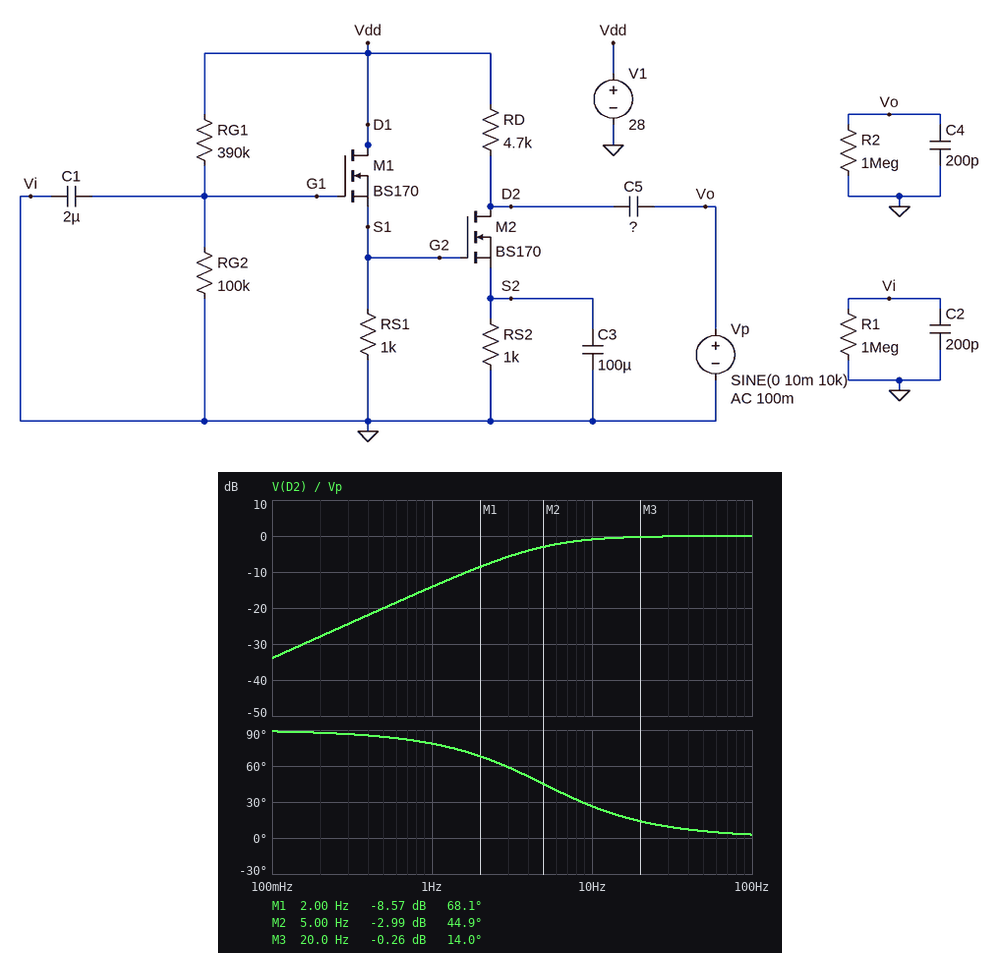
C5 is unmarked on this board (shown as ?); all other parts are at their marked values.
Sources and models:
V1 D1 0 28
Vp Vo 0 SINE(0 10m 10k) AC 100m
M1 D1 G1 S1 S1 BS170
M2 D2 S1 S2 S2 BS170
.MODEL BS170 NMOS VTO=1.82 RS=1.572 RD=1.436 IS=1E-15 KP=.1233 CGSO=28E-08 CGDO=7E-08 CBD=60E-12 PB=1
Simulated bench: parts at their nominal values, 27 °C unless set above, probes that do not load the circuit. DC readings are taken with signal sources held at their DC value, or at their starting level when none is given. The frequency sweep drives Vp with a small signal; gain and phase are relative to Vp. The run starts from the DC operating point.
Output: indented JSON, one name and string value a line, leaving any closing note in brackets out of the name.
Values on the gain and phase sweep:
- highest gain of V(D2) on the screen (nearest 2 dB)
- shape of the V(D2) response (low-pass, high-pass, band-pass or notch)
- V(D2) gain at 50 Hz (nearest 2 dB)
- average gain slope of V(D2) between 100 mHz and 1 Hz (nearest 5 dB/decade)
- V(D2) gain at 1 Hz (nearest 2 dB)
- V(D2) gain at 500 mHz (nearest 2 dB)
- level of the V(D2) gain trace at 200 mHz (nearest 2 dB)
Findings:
{
  "highest gain of V(D2) on the screen": "0 dB",
  "shape of the V(D2) response": "high-pass",
  "V(D2) gain at 50 Hz": "0 dB",
  "average gain slope of V(D2) between 100 mHz and 1 Hz": "20 dB/decade",
  "V(D2) gain at 1 Hz": "-14 dB",
  "V(D2) gain at 500 mHz": "-20 dB",
  "level of the V(D2) gain trace at 200 mHz": "-28 dB"
}
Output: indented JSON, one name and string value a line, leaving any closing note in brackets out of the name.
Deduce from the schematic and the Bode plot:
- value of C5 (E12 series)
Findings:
{
  "value of C5": "6.8 µF"
}
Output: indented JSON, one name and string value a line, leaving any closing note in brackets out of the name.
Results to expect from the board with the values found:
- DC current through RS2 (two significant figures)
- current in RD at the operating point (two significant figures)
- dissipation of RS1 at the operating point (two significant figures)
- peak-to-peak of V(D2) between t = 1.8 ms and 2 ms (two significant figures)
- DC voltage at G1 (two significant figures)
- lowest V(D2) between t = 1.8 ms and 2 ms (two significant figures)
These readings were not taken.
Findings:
{
  "DC current through RS2": "1.7 mA",
  "current in RD at the operating point": "1.7 mA",
  "dissipation of RS1 at the operating point": "13 mW",
  "peak-to-peak of V(D2) between t = 1.8 ms and 2 ms": "20 mV",
  "DC voltage at G1": "5.7 V",
  "lowest V(D2) between t = 1.8 ms and 2 ms": "20 V"
}
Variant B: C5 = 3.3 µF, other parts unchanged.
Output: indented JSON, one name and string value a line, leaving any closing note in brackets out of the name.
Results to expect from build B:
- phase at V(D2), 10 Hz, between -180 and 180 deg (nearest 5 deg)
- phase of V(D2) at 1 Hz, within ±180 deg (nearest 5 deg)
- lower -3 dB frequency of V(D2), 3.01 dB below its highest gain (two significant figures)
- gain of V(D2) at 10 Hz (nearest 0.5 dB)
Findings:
{
  "phase at V(D2), 10 Hz, between -180 and 180 deg": "45 deg",
  "phase of V(D2) at 1 Hz, within ±180 deg": "85 deg",
  "lower -3 dB frequency of V(D2), 3.01 dB below its highest gain": "10 Hz",
  "gain of V(D2) at 10 Hz": "-3.0 dB"
}
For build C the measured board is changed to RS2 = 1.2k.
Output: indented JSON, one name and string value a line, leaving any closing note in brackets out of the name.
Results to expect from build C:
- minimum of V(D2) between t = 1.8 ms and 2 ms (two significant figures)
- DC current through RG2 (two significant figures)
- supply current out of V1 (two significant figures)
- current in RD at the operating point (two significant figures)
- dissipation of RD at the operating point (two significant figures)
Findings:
{
  "minimum of V(D2) between t = 1.8 ms and 2 ms": "21 V",
  "DC current through RG2": "57 µA",
  "supply current out of V1": "5.1 mA",
  "current in RD at the operating point": "1.4 mA",
  "dissipation of RD at the operating point": "9.1 mW"
}
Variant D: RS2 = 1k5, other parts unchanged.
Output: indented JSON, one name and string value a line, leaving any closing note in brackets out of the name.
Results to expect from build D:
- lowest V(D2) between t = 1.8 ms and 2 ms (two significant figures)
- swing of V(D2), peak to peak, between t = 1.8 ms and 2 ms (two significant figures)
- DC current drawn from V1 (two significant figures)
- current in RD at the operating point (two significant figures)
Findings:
{
  "lowest V(D2) between t = 1.8 ms and 2 ms": "23 V",
  "swing of V(D2), peak to peak, between t = 1.8 ms and 2 ms": "20 mV",
  "DC current drawn from V1": "4.8 mA",
  "current in RD at the operating point": "1.1 mA"
}
